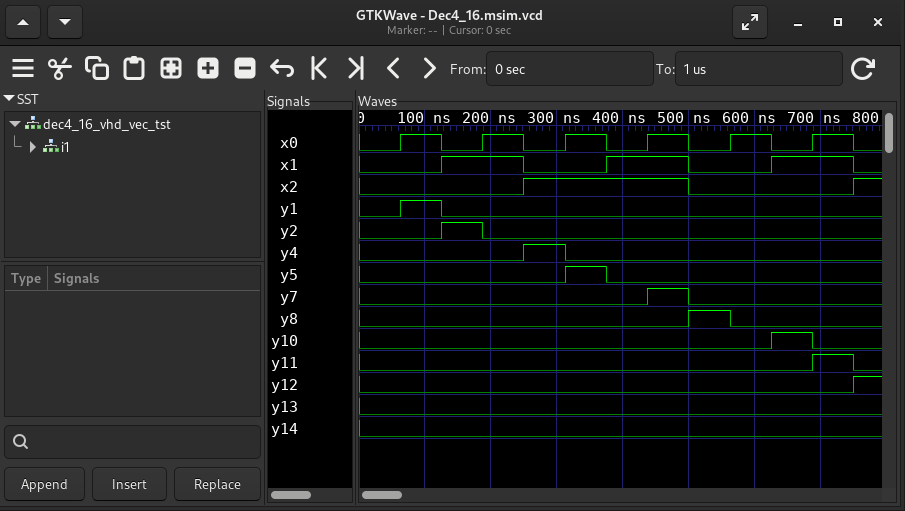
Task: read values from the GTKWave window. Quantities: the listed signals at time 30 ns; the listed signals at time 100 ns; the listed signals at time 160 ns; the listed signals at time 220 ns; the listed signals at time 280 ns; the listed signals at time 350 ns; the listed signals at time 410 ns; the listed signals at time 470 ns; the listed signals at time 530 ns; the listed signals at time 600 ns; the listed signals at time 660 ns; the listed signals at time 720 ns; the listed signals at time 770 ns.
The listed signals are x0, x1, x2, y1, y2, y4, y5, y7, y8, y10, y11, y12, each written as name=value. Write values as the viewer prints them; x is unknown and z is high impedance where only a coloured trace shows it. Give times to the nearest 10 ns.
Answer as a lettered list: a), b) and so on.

a) x0=0, x1=0, x2=0, y1=0, y2=0, y4=0, y5=0, y7=0, y8=0, y10=0, y11=0, y12=0
b) x0=1, x1=0, x2=0, y1=1, y2=0, y4=0, y5=0, y7=0, y8=0, y10=0, y11=0, y12=0
c) x0=0, x1=1, x2=0, y1=0, y2=1, y4=0, y5=0, y7=0, y8=0, y10=0, y11=0, y12=0
d) x0=1, x1=1, x2=0, y1=0, y2=0, y4=0, y5=0, y7=0, y8=0, y10=0, y11=0, y12=0
e) x0=0, x1=0, x2=1, y1=0, y2=0, y4=1, y5=0, y7=0, y8=0, y10=0, y11=0, y12=0
f) x0=1, x1=0, x2=1, y1=0, y2=0, y4=0, y5=1, y7=0, y8=0, y10=0, y11=0, y12=0
g) x0=0, x1=1, x2=1, y1=0, y2=0, y4=0, y5=0, y7=0, y8=0, y10=0, y11=0, y12=0
h) x0=1, x1=1, x2=1, y1=0, y2=0, y4=0, y5=0, y7=1, y8=0, y10=0, y11=0, y12=0
i) x0=0, x1=0, x2=0, y1=0, y2=0, y4=0, y5=0, y7=0, y8=1, y10=0, y11=0, y12=0
j) x0=1, x1=0, x2=0, y1=0, y2=0, y4=0, y5=0, y7=0, y8=0, y10=0, y11=0, y12=0
k) x0=0, x1=1, x2=0, y1=0, y2=0, y4=0, y5=0, y7=0, y8=0, y10=1, y11=0, y12=0
l) x0=1, x1=1, x2=0, y1=0, y2=0, y4=0, y5=0, y7=0, y8=0, y10=0, y11=1, y12=0
m) x0=0, x1=0, x2=1, y1=0, y2=0, y4=0, y5=0, y7=0, y8=0, y10=0, y11=0, y12=1
